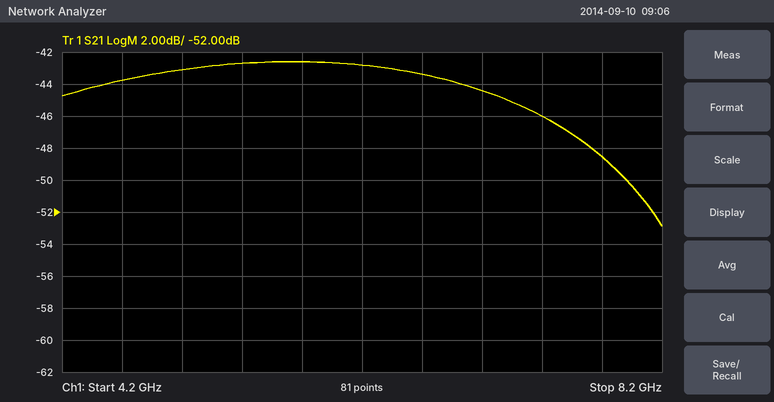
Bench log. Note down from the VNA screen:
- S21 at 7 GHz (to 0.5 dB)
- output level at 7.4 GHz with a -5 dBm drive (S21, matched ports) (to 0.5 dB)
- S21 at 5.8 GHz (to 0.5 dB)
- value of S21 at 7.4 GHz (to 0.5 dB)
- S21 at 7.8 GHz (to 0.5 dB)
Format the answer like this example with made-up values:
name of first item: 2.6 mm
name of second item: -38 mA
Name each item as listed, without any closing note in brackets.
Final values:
S21 at 7 GHz: -44.5 dB
output level at 7.4 GHz with a -5 dBm drive (S21, matched ports): -51.0 dBm
S21 at 5.8 GHz: -42.5 dB
value of S21 at 7.4 GHz: -46.0 dB
S21 at 7.8 GHz: -48.5 dB
